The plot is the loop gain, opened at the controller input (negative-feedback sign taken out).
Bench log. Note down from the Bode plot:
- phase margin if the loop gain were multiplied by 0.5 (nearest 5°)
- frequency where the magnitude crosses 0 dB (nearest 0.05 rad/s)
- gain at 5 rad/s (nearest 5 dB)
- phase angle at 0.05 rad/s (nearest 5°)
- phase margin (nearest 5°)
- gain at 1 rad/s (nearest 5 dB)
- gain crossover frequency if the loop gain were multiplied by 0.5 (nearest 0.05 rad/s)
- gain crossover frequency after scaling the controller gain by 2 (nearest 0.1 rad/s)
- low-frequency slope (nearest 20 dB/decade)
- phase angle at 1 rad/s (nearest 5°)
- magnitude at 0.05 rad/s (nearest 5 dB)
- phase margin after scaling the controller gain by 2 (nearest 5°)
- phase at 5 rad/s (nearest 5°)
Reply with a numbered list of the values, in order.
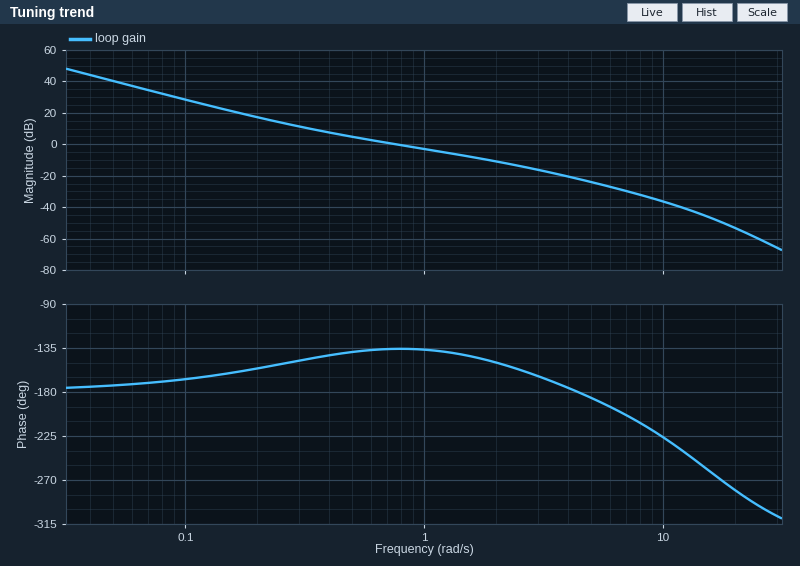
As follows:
1. 40°
2. 0.75 rad/s
3. -25 dB
4. -175°
5. 45°
6. -5 dB
7. 0.45 rad/s
8. 1.3 rad/s
9. -40 dB/decade
10. -135°
11. 40 dB
12. 40°
13. -185°
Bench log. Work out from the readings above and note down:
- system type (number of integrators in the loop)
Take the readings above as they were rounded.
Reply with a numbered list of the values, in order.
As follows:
1. 2
